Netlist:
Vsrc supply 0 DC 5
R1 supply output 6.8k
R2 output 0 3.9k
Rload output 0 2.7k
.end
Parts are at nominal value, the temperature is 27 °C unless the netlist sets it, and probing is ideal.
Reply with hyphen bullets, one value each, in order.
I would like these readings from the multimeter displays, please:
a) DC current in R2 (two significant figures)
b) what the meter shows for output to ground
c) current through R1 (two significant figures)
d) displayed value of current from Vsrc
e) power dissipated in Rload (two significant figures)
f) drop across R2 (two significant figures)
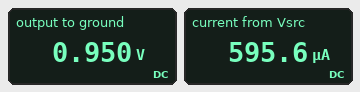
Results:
- 240 µA
- 0.950 V
- 600 µA
- 595.6 µA
- 330 µW
- 950 mV
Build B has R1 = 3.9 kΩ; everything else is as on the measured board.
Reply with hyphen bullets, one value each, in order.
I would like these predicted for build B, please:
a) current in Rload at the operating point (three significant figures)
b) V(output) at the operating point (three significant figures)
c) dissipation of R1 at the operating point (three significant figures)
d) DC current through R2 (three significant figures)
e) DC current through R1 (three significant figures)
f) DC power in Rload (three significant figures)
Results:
- 538 µA
- 1.45 V
- 3.23 mW
- 372 µA
- 910 µA
- 780 µW
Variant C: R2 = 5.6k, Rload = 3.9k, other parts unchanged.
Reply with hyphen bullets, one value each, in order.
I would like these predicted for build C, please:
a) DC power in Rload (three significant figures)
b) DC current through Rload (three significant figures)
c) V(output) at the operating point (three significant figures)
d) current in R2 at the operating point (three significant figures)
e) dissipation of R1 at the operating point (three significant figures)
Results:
- 409 µW
- 324 µA
- 1.26 V
- 226 µA
- 2.05 mW
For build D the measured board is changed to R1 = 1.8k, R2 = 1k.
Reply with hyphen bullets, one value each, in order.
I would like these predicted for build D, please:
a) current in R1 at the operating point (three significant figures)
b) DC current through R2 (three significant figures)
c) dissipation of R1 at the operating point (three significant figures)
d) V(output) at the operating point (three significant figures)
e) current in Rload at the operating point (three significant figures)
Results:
- 1.98 mA
- 1.44 mA
- 7.03 mW
- 1.44 V
- 534 µA
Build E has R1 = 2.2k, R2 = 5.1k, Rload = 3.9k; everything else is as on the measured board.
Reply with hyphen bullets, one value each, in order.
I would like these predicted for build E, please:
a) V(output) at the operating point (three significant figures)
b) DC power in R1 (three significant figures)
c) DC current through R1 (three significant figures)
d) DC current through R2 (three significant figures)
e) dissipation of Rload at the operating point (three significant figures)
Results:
- 2.51 V
- 2.83 mW
- 1.13 mA
- 491 µA
- 1.61 mW
